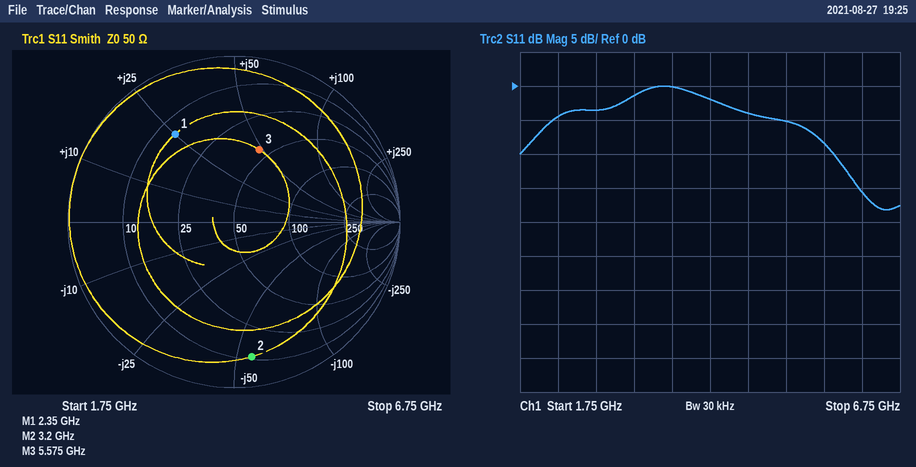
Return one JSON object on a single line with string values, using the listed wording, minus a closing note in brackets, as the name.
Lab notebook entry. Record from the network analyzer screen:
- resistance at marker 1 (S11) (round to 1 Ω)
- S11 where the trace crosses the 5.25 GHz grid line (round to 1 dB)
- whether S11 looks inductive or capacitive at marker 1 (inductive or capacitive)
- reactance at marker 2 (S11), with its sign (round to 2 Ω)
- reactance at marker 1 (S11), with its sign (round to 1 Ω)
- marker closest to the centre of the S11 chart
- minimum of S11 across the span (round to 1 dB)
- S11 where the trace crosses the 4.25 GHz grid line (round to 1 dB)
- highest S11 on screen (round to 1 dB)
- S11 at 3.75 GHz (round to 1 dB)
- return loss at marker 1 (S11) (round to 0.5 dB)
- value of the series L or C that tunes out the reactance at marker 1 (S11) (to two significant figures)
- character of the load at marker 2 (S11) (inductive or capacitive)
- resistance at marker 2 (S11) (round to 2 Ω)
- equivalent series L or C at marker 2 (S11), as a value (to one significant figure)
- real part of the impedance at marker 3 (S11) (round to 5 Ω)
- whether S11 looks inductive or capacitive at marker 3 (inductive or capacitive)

{"resistance at marker 1 (S11)": "14 Ω", "S11 where the trace crosses the 5.25 GHz grid line": "-5 dB", "whether S11 looks inductive or capacitive at marker 1": "inductive", "reactance at marker 2 (S11), with its sign": "-56 Ω", "reactance at marker 1 (S11), with its sign": "+25 Ω", "marker closest to the centre of the S11 chart": "marker 3", "minimum of S11 across the span": "-18 dB", "S11 where the trace crosses the 4.25 GHz grid line": "-2 dB", "highest S11 on screen": "0 dB", "S11 at 3.75 GHz": "0 dB", "return loss at marker 1 (S11)": "4.0 dB", "value of the series L or C that tunes out the reactance at marker 1 (S11)": "2.7 pF", "character of the load at marker 2 (S11)": "capacitive", "resistance at marker 2 (S11)": "12 Ω", "equivalent series L or C at marker 2 (S11), as a value": "900 fF", "real part of the impedance at marker 3 (S11)": "45 Ω", "whether S11 looks inductive or capacitive at marker 3": "inductive"}
